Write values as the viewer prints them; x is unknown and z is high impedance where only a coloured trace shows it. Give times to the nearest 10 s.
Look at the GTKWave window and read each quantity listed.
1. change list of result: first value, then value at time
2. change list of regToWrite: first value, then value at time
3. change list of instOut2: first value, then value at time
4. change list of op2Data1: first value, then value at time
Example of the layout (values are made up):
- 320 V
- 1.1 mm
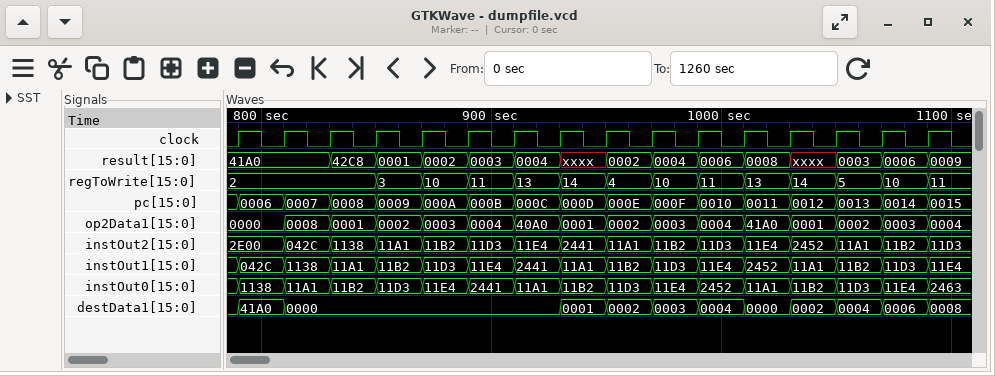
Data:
- 41A0, 42C8 at 830 s, 0001 at 850 s, 0002 at 870 s, 0003 at 890 s, 0004 at 910 s, xxxx at 930 s, 0002 at 950 s, 0004 at 970 s, 0006 at 990 s, 0008 at 1010 s, xxxx at 1030 s, 0003 at 1050 s, 0006 at 1070 s, 0009 at 1090 s
- 2, 3 at 850 s, 10 at 870 s, 11 at 890 s, 13 at 910 s, 14 at 930 s, 4 at 950 s, 10 at 970 s, 11 at 990 s, 13 at 1010 s, 14 at 1030 s, 5 at 1050 s, 10 at 1070 s, 11 at 1090 s
- 2E00, 042C at 810 s, 1138 at 830 s, 11A1 at 850 s, 11B2 at 870 s, 11D3 at 890 s, 11E4 at 910 s, 2441 at 930 s, 11A1 at 950 s, 11B2 at 970 s, 11D3 at 990 s, 11E4 at 1010 s, 2452 at 1030 s, 11A1 at 1050 s, 11B2 at 1070 s, 11D3 at 1090 s
- 0000, 0008 at 810 s, 0001 at 830 s, 0002 at 850 s, 0003 at 870 s, 0004 at 890 s, 40A0 at 910 s, 0001 at 930 s, 0002 at 950 s, 0003 at 970 s, 0004 at 990 s, 41A0 at 1010 s, 0001 at 1030 s, 0002 at 1050 s, 0003 at 1070 s, 0004 at 1090 s
